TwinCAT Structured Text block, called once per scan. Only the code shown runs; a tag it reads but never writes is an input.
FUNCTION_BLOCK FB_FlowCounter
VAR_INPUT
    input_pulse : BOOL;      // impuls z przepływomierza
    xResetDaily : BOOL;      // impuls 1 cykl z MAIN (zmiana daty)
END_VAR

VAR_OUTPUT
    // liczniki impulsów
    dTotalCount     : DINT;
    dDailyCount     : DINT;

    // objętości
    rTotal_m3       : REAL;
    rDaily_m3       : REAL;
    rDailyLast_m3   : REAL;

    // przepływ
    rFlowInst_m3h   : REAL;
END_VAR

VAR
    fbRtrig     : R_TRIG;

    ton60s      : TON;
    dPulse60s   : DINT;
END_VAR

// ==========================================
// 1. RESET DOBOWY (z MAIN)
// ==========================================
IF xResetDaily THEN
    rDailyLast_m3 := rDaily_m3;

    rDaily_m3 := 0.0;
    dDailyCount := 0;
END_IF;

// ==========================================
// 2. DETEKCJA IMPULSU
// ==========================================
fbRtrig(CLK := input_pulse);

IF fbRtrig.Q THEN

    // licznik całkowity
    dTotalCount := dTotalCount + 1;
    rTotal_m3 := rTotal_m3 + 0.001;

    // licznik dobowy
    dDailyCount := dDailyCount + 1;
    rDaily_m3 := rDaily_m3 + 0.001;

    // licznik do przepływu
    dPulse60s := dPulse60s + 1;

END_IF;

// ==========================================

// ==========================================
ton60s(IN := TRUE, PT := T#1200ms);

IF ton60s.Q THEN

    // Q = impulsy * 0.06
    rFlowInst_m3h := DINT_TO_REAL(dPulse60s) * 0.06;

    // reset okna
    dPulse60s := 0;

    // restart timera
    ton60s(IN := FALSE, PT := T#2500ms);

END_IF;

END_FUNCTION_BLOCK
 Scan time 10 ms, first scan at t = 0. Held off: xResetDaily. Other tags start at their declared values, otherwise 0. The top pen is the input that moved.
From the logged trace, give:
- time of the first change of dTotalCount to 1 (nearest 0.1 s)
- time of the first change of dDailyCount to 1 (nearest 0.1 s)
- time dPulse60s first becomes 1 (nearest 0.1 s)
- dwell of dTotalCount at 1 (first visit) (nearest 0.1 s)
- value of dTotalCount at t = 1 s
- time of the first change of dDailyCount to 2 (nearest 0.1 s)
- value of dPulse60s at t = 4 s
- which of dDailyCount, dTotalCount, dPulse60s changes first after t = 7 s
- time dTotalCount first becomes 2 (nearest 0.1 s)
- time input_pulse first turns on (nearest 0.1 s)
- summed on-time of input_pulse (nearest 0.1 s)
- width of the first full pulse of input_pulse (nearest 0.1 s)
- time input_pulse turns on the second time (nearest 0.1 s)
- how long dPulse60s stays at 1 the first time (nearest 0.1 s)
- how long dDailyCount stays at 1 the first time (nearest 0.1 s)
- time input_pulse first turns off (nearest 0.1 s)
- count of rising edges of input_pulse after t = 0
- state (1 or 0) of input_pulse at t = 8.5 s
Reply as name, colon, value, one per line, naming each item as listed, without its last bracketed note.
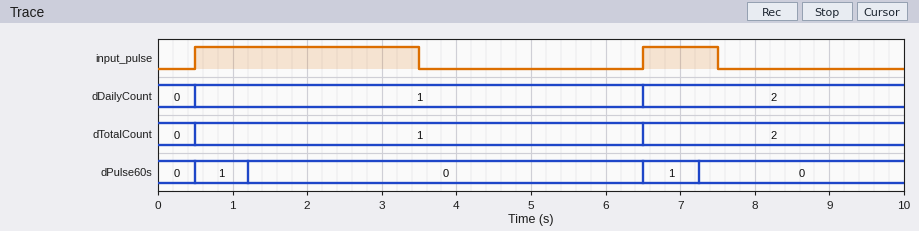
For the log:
time of the first change of dTotalCount to 1: 0.5 s
time of the first change of dDailyCount to 1: 0.5 s
time dPulse60s first becomes 1: 0.5 s
dwell of dTotalCount at 1 (first visit): 6.0 s
value of dTotalCount at t = 1 s: 1
time of the first change of dDailyCount to 2: 6.5 s
value of dPulse60s at t = 4 s: 0
which of dDailyCount, dTotalCount, dPulse60s changes first after t = 7 s: dPulse60s
time dTotalCount first becomes 2: 6.5 s
time input_pulse first turns on: 0.5 s
summed on-time of input_pulse: 4.0 s
width of the first full pulse of input_pulse: 3.0 s
time input_pulse turns on the second time: 6.5 s
how long dPulse60s stays at 1 the first time: 0.7 s
how long dDailyCount stays at 1 the first time: 6.0 s
time input_pulse first turns off: 3.5 s
count of rising edges of input_pulse after t = 0: 2
state (1 or 0) of input_pulse at t = 8.5 s: 0
